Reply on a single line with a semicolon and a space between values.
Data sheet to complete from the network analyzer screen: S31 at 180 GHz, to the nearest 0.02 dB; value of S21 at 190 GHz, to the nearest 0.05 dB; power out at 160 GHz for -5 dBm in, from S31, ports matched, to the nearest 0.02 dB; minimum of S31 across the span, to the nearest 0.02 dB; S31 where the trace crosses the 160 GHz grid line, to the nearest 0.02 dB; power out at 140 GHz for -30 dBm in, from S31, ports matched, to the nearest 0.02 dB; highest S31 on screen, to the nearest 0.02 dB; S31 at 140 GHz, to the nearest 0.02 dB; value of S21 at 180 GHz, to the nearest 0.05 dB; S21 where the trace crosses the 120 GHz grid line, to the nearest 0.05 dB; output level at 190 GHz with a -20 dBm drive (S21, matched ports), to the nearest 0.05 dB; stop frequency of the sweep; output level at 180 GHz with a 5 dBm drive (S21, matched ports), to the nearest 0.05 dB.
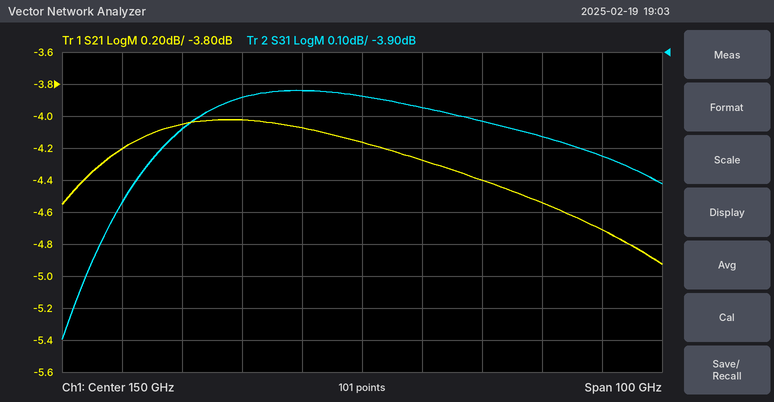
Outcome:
-4.16 dB; -4.70 dB; -9.08 dBm; -4.80 dB; -4.08 dB; -34.02 dBm; -4.02 dB; -4.02 dB; -4.55 dB; -4.05 dB; -24.70 dBm; 200 GHz; 0.45 dBm
